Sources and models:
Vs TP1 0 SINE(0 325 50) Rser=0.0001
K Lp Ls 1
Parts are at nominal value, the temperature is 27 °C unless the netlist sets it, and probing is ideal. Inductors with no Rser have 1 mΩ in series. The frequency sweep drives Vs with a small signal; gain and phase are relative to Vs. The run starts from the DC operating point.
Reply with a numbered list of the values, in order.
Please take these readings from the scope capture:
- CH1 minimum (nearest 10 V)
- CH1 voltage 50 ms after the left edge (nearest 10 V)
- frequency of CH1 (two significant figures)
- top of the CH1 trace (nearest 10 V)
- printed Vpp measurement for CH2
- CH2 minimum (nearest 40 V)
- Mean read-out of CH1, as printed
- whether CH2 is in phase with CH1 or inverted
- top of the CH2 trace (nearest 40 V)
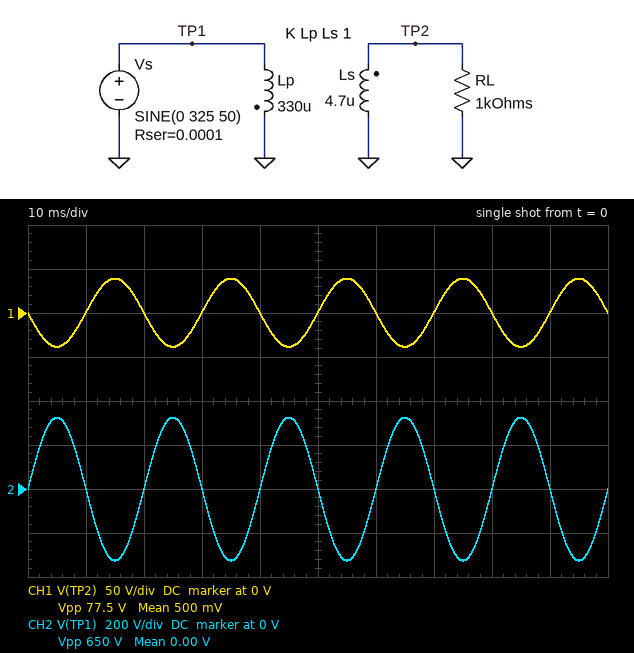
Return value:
1. -40 V
2. 0 V
3. 50 Hz
4. 40 V
5. 650 V
6. -320 V
7. 500 mV
8. inverted
9. 320 V
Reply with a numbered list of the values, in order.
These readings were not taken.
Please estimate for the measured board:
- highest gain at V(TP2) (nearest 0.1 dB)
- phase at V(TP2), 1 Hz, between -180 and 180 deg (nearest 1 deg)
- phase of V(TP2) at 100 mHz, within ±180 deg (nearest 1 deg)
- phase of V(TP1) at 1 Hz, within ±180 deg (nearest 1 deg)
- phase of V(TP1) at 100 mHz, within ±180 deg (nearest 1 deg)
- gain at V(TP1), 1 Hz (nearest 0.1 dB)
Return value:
1. -18.5 dB
2. -152 deg
3. -101 deg
4. 2 deg
5. 1 deg
6. -0.2 dB
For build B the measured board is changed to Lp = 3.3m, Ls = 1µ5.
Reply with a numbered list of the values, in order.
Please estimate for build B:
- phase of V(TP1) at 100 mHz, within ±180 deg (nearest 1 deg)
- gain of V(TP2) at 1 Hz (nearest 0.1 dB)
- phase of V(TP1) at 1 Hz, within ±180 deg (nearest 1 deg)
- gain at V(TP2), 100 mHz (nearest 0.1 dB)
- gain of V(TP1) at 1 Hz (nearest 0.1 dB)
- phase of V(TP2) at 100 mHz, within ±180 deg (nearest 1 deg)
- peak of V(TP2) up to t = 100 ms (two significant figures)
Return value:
1. 2 deg
2. -33.4 dB
3. 0 deg
4. -34.5 dB
5. 0 dB
6. -152 deg
7. 6.9 V
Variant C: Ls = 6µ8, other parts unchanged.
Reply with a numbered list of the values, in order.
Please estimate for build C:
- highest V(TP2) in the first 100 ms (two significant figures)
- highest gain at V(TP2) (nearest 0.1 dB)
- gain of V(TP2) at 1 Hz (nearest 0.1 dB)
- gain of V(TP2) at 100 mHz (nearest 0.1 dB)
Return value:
1. 47 V
2. -16.9 dB
3. -17.9 dB
4. -31.5 dB
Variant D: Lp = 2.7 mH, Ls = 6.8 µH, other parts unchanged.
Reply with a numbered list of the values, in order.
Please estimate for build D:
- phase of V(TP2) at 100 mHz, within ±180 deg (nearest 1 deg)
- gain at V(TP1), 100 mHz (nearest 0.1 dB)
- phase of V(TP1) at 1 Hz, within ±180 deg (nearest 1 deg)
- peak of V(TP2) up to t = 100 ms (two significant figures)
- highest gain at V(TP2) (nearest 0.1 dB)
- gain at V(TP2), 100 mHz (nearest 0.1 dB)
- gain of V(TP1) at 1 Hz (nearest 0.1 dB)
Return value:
1. -147 deg
2. -0.2 dB
3. 0 deg
4. 16 V
5. -26.0 dB
6. -27.5 dB
7. 0 dB
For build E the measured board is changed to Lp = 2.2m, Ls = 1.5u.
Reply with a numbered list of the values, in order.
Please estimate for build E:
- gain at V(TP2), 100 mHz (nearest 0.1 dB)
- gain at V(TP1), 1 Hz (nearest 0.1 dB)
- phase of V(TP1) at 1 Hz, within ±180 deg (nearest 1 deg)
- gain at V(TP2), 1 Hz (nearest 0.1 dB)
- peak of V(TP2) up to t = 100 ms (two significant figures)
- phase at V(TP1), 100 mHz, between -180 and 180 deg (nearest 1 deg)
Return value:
1. -33.8 dB
2. 0 dB
3. 0 deg
4. -31.7 dB
5. 8.5 V
6. 3 deg
